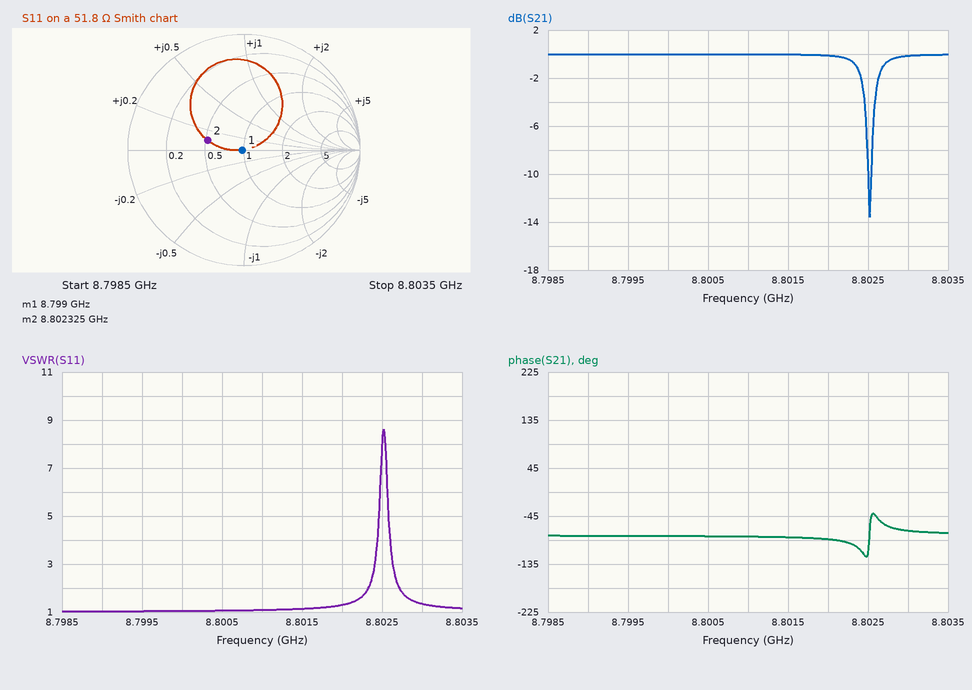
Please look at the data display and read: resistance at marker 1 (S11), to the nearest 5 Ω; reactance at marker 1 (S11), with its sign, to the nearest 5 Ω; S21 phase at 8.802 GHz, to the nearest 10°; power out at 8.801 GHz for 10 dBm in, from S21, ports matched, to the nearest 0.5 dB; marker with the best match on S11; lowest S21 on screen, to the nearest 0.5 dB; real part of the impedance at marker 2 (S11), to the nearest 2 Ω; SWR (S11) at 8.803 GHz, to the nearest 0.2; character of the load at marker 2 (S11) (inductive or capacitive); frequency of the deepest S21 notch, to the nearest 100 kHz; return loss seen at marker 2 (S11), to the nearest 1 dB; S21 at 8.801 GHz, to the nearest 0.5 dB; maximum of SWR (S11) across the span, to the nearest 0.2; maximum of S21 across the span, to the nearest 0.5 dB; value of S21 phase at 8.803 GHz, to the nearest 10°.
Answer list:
50 Ω
0 Ω
-90°
10.0 dBm
marker 1
-13.5 dB
26 Ω
1.4
inductive
8.8025 GHz
10 dB
0.0 dB
8.6
0.0 dB
-70°
